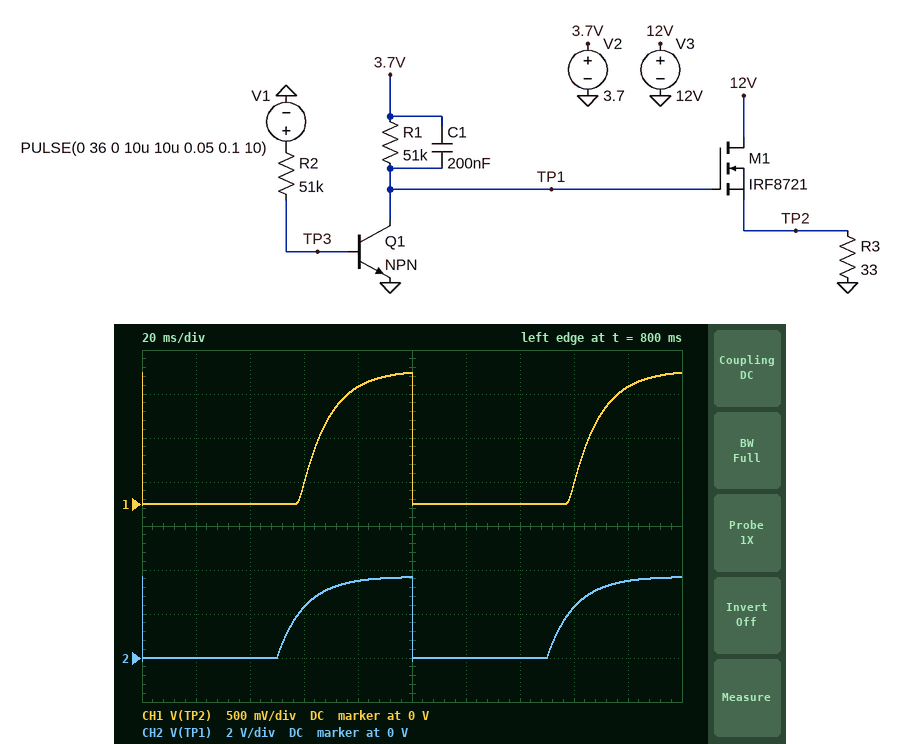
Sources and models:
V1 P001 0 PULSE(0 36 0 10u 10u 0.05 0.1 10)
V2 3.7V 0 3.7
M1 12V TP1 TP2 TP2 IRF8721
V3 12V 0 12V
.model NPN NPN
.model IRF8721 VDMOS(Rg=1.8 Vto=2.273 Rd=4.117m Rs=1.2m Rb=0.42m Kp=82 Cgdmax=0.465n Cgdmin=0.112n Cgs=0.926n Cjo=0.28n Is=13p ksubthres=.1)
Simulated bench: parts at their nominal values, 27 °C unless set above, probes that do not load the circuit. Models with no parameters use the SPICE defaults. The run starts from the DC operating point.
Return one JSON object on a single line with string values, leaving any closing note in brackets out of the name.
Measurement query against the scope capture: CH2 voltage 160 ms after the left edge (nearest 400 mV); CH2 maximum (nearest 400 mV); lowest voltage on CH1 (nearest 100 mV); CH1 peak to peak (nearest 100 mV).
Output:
{"CH2 voltage 160 ms after the left edge": "2.4 V", "CH2 maximum": "3.6 V", "lowest voltage on CH1": "0 V", "CH1 peak to peak": "1.5 V"}
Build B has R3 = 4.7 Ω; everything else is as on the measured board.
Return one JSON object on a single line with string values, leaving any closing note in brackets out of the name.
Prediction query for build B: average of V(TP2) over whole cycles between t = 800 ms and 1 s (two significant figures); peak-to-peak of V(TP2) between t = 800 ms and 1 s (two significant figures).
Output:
{"average of V(TP2) over whole cycles between t = 800 ms and 1 s": "430 mV", "peak-to-peak of V(TP2) between t = 800 ms and 1 s": "1.4 V"}
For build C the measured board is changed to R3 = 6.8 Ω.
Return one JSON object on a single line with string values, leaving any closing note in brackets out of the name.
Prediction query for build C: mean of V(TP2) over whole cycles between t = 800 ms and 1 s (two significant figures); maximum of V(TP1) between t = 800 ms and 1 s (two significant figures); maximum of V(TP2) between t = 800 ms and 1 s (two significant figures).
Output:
{"mean of V(TP2) over whole cycles between t = 800 ms and 1 s": "440 mV", "maximum of V(TP1) between t = 800 ms and 1 s": "3.7 V", "maximum of V(TP2) between t = 800 ms and 1 s": "1.4 V"}
